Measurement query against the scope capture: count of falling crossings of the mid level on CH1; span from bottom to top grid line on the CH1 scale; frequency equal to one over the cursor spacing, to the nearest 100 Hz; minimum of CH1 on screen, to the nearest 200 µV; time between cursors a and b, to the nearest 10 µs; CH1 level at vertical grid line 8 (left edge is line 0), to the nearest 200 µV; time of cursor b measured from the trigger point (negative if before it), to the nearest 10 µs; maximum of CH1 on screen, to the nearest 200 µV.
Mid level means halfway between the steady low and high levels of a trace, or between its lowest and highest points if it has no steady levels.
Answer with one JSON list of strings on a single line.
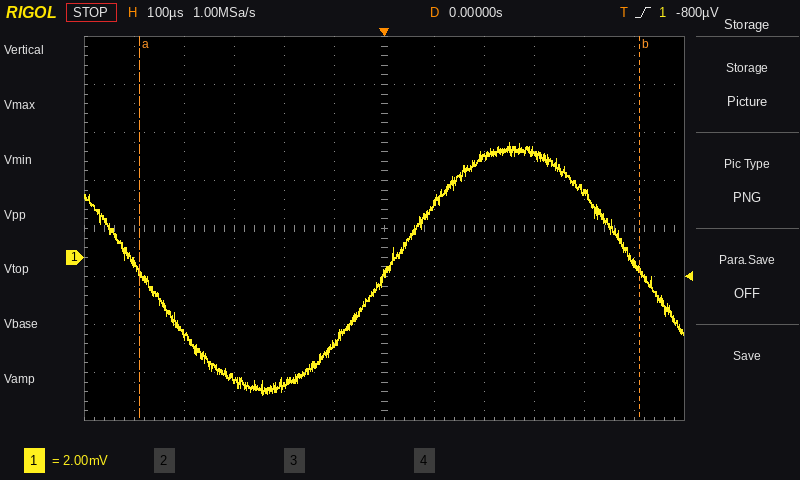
["2", "16 mV", "1.0 kHz", "-5.8 mV", "1.00 ms", "4.2 mV", "+510 µs", "4.8 mV"]
